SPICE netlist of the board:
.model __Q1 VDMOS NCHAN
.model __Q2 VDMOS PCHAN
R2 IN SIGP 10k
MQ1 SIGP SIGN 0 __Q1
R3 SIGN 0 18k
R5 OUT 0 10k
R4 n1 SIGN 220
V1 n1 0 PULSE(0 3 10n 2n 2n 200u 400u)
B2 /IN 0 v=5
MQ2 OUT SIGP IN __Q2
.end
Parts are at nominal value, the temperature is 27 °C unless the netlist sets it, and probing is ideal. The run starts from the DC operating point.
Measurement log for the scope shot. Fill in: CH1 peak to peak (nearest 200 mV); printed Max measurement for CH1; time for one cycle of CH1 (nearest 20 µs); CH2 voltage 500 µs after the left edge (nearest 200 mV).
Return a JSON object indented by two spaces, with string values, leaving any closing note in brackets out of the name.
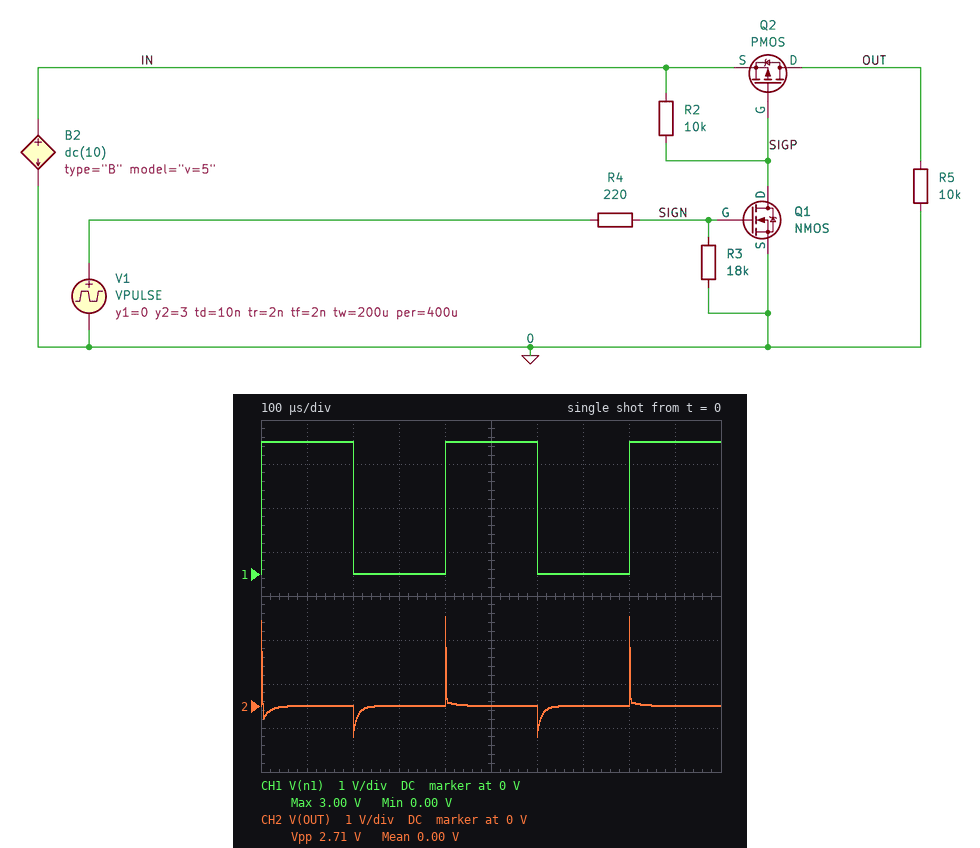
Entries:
{
  "CH1 peak to peak": "3.0 V",
  "printed Max measurement for CH1": "3.00 V",
  "time for one cycle of CH1": "400 µs",
  "CH2 voltage 500 µs after the left edge": "0 V"
}
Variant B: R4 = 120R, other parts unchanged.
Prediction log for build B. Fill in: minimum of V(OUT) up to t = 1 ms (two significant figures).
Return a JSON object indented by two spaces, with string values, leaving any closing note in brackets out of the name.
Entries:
{
  "minimum of V(OUT) up to t = 1 ms": "-710 mV"
}
